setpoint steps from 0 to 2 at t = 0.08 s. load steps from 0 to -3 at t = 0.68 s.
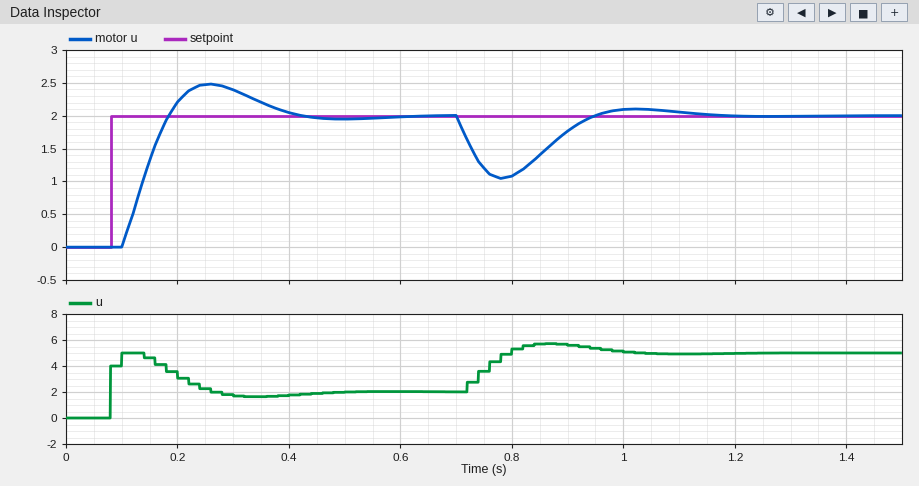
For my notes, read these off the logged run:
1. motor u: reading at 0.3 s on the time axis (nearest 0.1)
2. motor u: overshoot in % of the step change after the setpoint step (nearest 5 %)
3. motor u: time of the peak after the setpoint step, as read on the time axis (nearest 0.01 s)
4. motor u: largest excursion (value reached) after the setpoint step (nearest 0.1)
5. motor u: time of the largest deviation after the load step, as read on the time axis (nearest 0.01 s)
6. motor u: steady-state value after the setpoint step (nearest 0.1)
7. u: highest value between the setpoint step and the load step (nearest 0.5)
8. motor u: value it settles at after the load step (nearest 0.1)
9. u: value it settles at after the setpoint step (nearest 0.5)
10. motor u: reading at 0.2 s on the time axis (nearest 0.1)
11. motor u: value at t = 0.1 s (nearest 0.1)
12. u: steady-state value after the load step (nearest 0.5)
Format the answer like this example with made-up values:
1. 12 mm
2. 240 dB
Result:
1. 2.4
2. 25 %
3. 0.26 s
4. 2.5
5. 0.78 s
6. 2.0
7. 5.0
8. 2.0
9. 2.0
10. 2.2
11. 0.0
12. 5.0
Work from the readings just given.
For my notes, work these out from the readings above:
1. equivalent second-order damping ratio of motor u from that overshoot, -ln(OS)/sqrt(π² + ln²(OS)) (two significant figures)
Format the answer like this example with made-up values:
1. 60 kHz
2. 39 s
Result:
1. 0.40
